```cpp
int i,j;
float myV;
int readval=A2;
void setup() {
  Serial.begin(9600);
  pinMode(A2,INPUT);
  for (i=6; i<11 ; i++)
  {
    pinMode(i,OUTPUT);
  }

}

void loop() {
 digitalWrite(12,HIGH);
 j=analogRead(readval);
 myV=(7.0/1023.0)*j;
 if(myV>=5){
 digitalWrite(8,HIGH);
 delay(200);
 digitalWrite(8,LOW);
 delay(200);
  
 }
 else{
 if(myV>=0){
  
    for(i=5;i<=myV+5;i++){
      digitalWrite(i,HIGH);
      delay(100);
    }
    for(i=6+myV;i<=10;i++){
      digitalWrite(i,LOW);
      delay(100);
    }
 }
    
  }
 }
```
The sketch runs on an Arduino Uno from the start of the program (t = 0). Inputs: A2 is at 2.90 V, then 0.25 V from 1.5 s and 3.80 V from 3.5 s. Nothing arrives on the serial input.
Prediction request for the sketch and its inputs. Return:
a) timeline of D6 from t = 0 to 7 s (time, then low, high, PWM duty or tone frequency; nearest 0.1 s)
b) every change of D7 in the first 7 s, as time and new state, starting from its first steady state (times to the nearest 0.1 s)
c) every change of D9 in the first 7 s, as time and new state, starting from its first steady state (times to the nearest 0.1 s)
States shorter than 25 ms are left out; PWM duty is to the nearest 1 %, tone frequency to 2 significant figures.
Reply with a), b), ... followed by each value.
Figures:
a) 0 s low; 0.1 s high; 1.9 s low
b) 0 s low; 0.2 s high; 2 s low
c) 0 s low; 0.4 s high; 2.2 s low
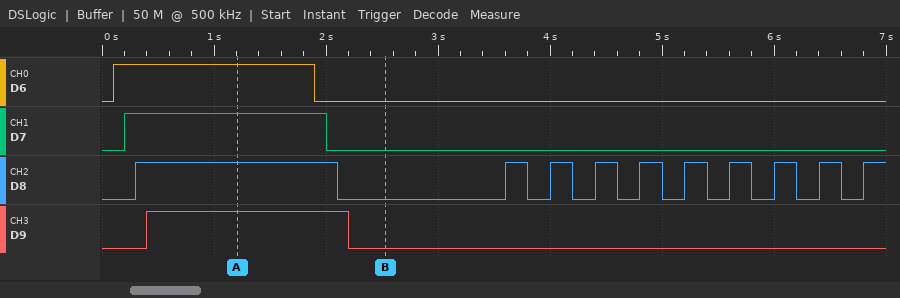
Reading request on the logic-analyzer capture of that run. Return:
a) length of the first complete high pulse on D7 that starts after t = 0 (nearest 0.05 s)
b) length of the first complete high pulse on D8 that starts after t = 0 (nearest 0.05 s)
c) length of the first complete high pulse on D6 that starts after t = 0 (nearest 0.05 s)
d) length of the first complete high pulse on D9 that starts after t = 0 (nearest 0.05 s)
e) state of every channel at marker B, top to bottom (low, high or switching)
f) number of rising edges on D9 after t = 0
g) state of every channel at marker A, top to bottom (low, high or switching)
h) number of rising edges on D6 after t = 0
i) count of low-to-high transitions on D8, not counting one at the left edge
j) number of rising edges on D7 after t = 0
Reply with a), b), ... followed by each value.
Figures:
a) 1.80 s
b) 1.80 s
c) 1.80 s
d) 1.80 s
e) D6 low, D7 low, D8 low, D9 low
f) 1
g) D6 high, D7 high, D8 high, D9 high
h) 1
i) 10
j) 1
